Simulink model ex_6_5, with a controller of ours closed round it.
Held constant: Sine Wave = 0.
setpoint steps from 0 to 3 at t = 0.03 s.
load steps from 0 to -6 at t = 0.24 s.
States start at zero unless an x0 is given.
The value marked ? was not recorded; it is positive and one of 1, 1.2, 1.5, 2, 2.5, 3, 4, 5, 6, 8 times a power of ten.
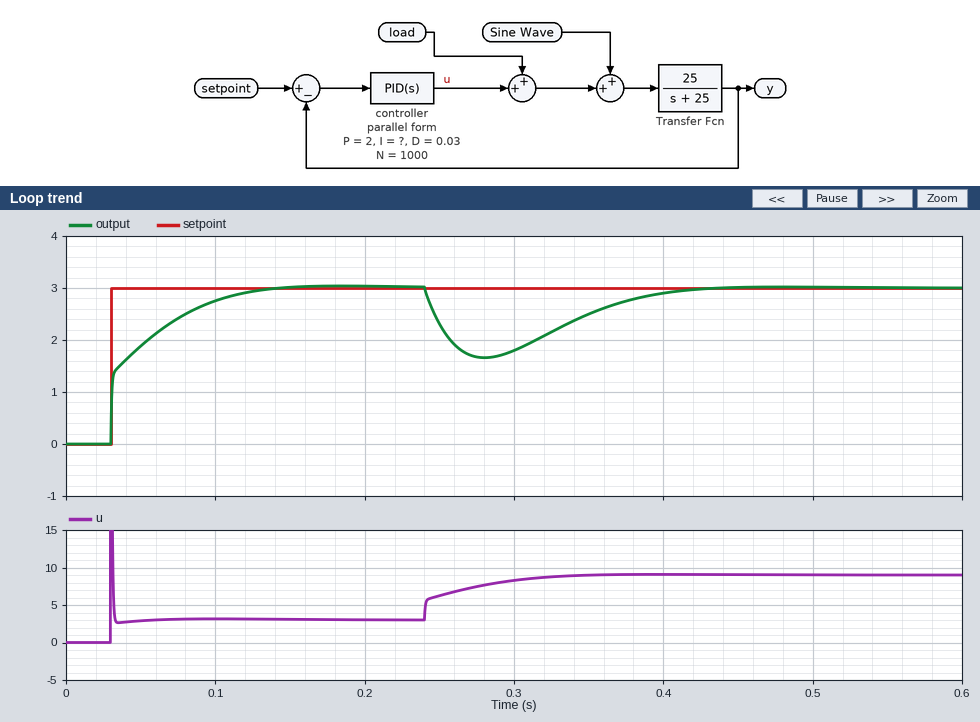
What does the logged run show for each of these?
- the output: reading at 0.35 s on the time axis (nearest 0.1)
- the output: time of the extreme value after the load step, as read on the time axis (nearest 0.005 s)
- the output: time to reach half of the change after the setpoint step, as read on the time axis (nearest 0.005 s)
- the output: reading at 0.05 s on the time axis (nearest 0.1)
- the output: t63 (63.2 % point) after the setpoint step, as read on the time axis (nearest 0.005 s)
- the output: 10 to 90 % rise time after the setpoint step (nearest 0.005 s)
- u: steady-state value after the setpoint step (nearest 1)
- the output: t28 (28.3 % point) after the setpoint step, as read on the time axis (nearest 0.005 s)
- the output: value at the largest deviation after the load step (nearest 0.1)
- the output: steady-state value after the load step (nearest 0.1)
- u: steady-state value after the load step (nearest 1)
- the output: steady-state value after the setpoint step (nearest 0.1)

2.5
0.280 s
0.035 s
1.9
0.050 s
0.065 s
3
0.030 s
1.7
3.0
9
3.0
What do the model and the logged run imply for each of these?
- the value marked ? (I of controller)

50
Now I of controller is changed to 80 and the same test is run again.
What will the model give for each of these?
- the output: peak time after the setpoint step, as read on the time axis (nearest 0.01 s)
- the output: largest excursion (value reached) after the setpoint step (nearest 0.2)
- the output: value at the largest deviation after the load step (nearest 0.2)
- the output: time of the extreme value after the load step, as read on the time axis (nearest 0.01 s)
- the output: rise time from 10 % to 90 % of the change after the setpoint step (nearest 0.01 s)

0.13 s
3.2
1.8
0.27 s
0.05 s
